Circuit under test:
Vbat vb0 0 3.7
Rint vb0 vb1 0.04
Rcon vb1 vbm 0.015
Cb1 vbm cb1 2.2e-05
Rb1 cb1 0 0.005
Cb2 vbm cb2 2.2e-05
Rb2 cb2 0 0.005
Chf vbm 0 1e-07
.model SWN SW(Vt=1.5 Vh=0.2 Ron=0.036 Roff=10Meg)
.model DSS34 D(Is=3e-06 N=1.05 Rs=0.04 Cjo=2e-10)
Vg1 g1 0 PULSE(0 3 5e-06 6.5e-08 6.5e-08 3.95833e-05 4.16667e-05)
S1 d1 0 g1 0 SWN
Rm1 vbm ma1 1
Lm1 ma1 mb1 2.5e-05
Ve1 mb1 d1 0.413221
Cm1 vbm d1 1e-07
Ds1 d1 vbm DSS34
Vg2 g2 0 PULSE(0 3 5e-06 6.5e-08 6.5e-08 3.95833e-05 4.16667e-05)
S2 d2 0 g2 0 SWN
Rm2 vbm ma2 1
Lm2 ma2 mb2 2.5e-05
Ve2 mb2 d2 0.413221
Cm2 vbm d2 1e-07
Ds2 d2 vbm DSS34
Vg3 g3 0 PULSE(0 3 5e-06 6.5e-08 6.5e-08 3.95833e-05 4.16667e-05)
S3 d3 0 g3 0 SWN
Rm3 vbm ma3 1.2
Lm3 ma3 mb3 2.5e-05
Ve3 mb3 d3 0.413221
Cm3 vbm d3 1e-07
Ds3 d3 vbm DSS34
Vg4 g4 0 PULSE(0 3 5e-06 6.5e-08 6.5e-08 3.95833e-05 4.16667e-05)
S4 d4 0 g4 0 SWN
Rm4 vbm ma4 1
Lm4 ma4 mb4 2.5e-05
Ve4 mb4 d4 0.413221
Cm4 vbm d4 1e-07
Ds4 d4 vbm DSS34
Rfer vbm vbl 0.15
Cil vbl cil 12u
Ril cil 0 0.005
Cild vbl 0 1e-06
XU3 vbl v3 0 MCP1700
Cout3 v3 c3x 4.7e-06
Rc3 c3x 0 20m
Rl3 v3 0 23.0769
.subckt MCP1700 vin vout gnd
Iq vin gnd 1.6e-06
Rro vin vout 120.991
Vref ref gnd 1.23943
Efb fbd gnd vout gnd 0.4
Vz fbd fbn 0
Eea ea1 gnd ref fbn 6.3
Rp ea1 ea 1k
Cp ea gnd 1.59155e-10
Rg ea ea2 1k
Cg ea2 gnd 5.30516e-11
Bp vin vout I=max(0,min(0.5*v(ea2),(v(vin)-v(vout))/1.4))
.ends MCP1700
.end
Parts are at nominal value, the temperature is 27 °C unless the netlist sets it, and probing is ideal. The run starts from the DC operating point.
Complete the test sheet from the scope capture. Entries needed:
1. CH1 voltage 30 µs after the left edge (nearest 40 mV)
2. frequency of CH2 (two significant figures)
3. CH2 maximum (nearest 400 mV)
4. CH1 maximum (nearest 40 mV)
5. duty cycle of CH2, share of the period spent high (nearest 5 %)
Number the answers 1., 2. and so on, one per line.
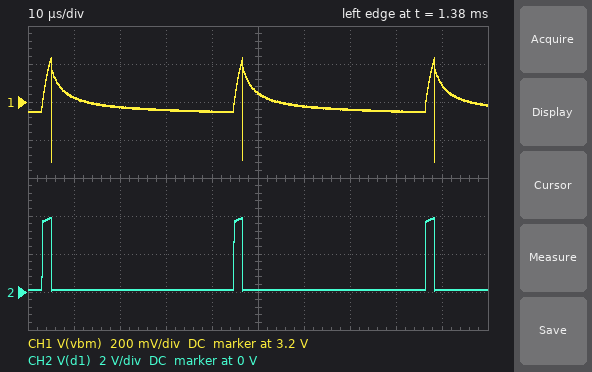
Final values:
1. 3.16 V
2. 24 kHz
3. 4.0 V
4. 3.44 V
5. 5 %
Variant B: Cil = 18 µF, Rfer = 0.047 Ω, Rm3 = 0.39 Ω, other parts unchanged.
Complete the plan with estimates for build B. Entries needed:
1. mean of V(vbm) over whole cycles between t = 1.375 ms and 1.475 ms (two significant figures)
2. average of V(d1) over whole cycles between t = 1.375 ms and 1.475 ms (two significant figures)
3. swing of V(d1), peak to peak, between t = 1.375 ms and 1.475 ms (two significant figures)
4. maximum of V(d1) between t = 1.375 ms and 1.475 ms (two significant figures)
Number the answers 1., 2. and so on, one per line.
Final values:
1. 3.0 V
2. 250 mV
3. 3.7 V
4. 3.8 V
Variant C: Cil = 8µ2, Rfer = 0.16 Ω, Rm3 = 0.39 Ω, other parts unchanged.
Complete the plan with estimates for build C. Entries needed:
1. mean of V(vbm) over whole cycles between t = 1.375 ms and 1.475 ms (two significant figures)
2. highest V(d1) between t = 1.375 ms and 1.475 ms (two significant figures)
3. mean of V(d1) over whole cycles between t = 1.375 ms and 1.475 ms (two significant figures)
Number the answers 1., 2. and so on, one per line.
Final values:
1. 3.0 V
2. 3.8 V
3. 250 mV
